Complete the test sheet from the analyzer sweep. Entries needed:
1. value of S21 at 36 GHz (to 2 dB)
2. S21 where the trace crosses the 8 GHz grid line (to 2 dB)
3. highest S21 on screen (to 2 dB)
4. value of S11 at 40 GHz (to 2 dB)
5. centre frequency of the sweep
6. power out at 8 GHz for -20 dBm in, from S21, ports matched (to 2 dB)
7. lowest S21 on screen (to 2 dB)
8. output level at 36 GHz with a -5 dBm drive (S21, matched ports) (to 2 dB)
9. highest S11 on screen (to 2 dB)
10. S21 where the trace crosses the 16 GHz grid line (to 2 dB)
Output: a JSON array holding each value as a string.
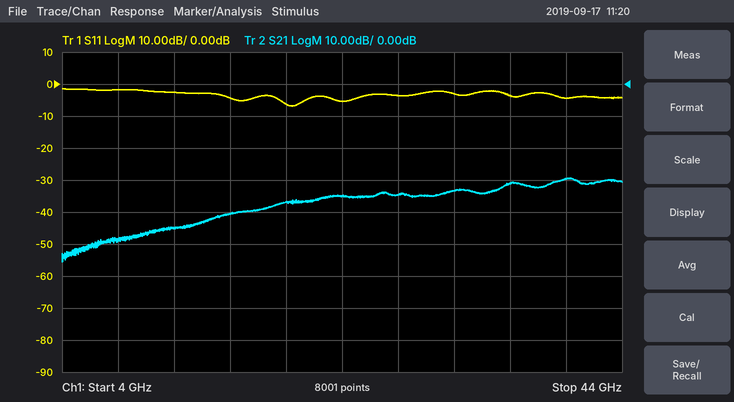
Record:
["-32 dB", "-48 dB", "-30 dB", "-4 dB", "24 GHz", "-68 dBm", "-56 dB", "-36 dBm", "-2 dB", "-40 dB"]
